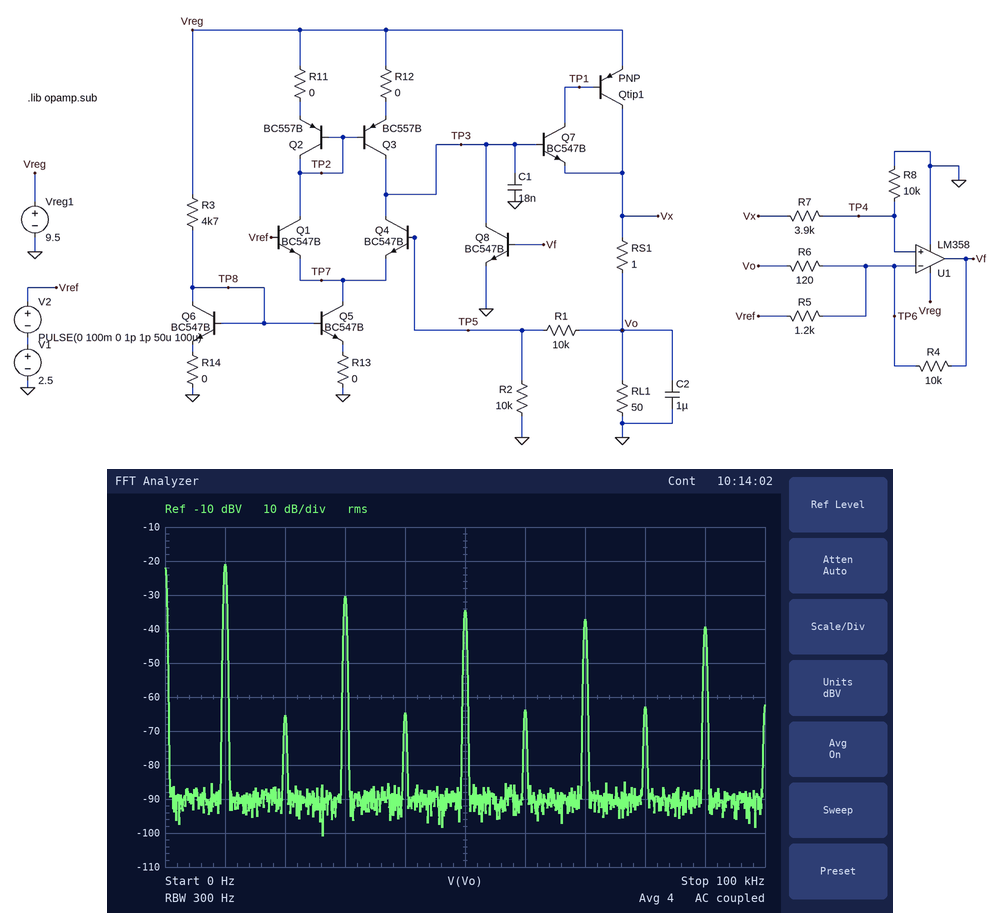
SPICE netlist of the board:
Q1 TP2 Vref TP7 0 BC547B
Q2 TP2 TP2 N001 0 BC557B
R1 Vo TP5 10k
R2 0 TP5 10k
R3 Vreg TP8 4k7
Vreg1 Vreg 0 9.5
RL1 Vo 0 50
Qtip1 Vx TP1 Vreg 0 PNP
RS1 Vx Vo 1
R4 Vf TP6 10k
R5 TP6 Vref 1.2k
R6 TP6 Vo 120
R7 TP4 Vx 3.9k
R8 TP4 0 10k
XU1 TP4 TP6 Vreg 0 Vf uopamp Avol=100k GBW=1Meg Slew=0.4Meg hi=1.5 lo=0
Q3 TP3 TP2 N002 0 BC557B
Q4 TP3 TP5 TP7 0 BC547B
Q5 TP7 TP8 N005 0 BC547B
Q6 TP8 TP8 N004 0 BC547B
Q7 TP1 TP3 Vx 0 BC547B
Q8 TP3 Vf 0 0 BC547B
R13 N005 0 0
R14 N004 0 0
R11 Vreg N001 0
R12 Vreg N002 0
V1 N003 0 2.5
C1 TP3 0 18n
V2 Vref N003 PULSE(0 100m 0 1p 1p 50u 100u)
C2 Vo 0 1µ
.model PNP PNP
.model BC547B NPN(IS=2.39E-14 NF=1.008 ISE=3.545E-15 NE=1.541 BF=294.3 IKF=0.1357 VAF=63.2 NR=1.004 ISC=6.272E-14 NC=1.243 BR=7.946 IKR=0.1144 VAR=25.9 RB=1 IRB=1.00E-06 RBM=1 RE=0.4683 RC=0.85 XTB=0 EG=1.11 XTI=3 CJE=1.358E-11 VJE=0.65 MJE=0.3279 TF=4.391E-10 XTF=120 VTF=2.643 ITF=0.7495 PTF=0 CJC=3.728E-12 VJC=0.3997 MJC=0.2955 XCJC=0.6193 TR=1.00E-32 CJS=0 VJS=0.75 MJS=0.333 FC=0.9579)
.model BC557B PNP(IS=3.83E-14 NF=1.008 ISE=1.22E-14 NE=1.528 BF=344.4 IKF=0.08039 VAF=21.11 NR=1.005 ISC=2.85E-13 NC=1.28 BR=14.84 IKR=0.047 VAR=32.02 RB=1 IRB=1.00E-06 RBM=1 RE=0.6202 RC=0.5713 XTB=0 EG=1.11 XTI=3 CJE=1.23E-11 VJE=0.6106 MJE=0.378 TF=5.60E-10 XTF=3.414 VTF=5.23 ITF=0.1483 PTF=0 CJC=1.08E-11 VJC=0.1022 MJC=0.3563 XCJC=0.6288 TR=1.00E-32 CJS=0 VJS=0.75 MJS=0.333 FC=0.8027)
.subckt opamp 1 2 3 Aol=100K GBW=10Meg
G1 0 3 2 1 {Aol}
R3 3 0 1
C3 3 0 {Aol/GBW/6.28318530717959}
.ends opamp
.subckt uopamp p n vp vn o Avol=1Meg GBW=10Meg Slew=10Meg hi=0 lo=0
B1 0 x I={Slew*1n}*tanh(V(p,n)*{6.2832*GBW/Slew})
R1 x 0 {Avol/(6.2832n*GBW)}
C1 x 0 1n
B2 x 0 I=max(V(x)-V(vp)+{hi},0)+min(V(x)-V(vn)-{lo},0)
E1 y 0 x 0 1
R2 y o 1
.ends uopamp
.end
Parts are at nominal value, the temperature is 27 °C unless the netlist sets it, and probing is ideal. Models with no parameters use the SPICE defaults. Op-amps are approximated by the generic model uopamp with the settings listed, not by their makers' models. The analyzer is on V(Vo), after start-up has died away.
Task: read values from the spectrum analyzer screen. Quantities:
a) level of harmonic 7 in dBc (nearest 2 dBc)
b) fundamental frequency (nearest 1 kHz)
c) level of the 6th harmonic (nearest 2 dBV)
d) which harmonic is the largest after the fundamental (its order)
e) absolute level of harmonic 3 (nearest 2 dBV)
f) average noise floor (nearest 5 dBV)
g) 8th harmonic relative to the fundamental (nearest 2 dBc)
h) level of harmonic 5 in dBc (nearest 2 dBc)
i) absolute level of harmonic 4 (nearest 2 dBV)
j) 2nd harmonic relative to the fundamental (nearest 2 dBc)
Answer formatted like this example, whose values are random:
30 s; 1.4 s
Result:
-16 dBc; 10 kHz; -64 dBV; 3; -30 dBV; -90 dBV; -42 dBc; -14 dBc; -64 dBV; -44 dBc
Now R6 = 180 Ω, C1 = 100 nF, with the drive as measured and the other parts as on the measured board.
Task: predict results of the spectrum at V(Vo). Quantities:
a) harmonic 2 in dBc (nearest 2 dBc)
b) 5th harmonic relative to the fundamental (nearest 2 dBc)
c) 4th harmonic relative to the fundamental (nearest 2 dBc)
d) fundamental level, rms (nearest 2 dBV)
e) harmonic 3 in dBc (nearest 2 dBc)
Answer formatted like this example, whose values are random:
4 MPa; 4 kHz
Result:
-36 dBc; -22 dBc; -42 dBc; -22 dBV; -14 dBc
